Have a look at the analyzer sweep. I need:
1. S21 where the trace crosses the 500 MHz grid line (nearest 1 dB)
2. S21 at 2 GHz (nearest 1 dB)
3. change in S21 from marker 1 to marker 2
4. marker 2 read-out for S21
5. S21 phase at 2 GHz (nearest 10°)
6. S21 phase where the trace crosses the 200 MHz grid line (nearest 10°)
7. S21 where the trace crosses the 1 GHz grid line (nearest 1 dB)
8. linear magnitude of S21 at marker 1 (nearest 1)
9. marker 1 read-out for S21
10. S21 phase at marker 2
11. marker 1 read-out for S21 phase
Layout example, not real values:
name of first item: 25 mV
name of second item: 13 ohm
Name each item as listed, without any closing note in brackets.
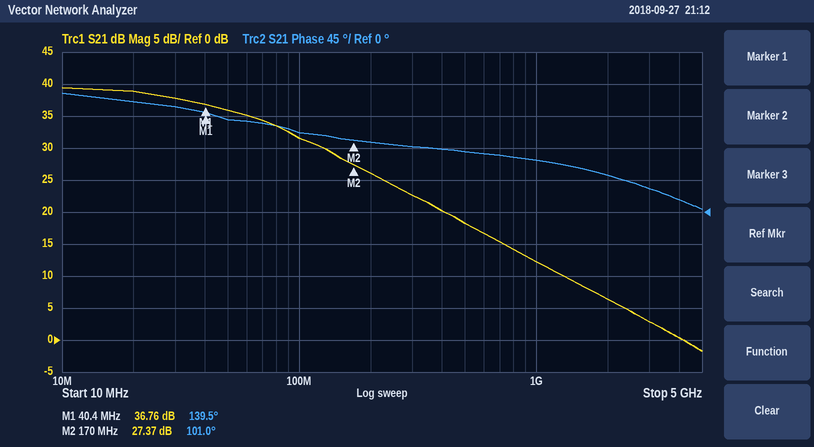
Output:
S21 where the trace crosses the 500 MHz grid line: 18 dB
S21 at 2 GHz: 6 dB
change in S21 from marker 1 to marker 2: -9.39 dB
marker 2 read-out for S21: 27.37 dB
S21 phase at 2 GHz: 50°
S21 phase where the trace crosses the 200 MHz grid line: 100°
S21 where the trace crosses the 1 GHz grid line: 12 dB
linear magnitude of S21 at marker 1: 69
marker 1 read-out for S21: 36.76 dB
S21 phase at marker 2: 101.0°
marker 1 read-out for S21 phase: 139.5°
